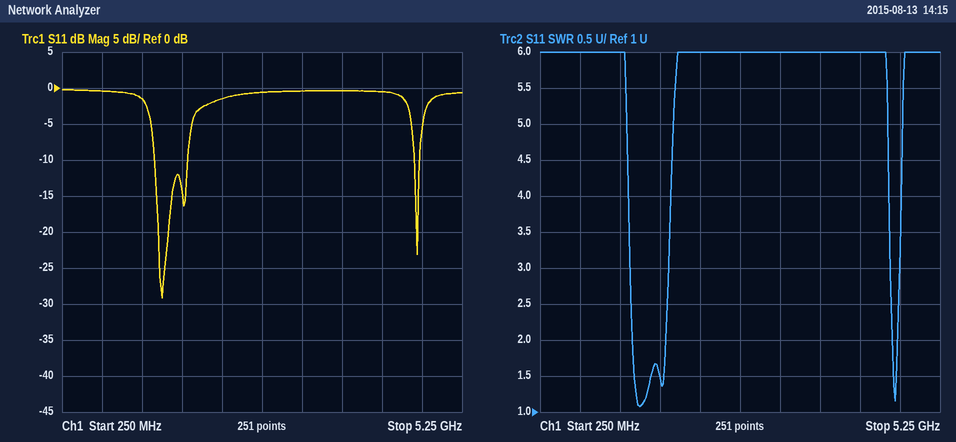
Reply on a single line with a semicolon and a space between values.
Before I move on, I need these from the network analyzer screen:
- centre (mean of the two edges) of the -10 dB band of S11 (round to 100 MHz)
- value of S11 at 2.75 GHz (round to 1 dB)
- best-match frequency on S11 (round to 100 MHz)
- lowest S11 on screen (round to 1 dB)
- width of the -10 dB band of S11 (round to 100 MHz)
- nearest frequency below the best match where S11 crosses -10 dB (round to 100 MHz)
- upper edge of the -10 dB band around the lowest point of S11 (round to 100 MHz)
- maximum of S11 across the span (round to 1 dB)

1.6 GHz; -1 dB; 1.5 GHz; -29 dB; 400 MHz; 1.4 GHz; 1.8 GHz; 0 dB
